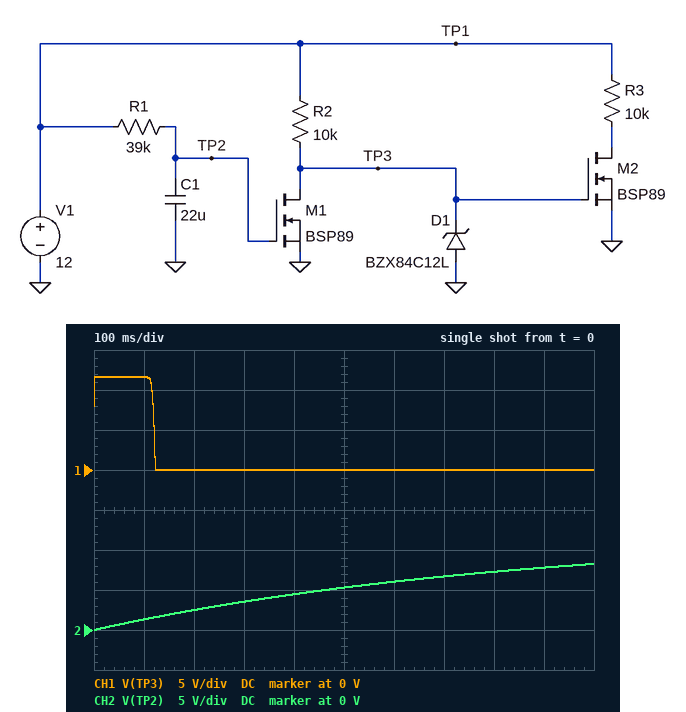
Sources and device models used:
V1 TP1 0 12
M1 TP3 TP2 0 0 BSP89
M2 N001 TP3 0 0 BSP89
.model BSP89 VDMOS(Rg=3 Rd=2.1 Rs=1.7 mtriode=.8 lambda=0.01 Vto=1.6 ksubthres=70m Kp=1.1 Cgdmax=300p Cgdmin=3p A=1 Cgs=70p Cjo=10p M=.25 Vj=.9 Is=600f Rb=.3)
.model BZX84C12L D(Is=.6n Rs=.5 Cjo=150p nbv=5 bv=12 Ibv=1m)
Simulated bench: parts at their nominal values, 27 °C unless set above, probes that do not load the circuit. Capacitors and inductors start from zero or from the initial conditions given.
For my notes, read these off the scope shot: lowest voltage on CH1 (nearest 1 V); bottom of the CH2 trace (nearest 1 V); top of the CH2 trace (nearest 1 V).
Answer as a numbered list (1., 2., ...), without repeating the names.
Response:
1. 0 V
2. 0 V
3. 8 V
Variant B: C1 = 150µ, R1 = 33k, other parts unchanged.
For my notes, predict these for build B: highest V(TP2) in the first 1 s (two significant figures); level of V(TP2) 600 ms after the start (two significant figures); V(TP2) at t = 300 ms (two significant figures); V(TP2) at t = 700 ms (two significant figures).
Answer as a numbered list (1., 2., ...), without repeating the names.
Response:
1. 2.2 V
2. 1.4 V
3. 710 mV
4. 1.6 V
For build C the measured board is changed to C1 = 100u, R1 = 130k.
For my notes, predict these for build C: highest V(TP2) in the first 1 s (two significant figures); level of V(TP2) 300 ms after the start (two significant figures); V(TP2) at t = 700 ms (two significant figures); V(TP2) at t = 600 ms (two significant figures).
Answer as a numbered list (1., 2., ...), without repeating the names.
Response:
1. 890 mV
2. 270 mV
3. 630 mV
4. 540 mV
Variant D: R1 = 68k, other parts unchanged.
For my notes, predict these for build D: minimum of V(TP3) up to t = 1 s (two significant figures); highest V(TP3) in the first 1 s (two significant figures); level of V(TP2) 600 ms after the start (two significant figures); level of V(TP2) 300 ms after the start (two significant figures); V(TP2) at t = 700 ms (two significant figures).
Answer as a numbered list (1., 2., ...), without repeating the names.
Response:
1. 4.9 mV
2. 12 V
3. 4.0 V
4. 2.2 V
5. 4.5 V
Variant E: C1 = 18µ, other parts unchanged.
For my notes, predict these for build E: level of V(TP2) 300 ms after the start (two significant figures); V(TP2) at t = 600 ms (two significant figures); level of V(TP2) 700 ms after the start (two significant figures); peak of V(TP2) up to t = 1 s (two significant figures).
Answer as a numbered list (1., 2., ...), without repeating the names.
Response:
1. 4.2 V
2. 6.9 V
3. 7.6 V
4. 9.1 V
